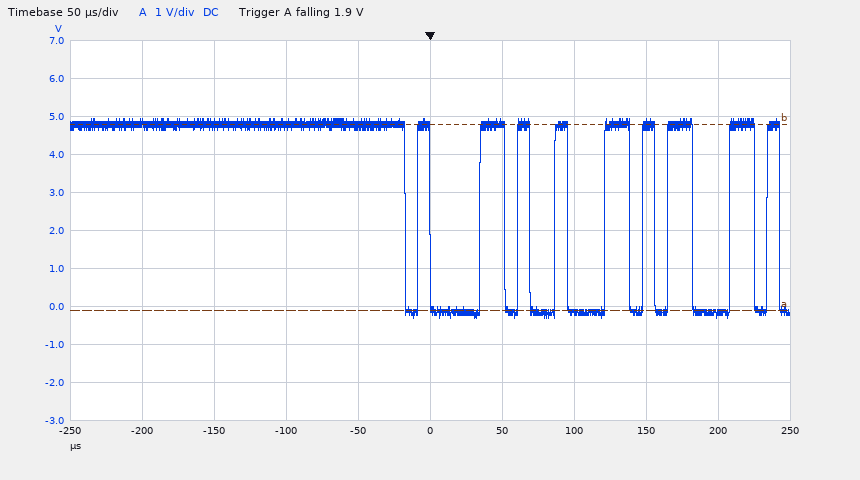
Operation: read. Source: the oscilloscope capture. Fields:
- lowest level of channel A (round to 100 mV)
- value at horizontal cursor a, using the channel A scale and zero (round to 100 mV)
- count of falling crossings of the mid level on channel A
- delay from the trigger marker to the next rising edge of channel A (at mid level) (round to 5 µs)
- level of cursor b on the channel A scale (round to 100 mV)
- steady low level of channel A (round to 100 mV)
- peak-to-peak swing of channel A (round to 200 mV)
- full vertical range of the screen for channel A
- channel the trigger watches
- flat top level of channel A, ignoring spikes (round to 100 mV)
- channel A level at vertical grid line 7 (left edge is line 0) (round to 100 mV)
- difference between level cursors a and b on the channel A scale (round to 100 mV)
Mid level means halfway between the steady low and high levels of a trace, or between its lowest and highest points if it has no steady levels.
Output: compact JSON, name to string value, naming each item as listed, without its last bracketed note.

{"lowest level of channel A": "-300 mV", "value at horizontal cursor a, using the channel A scale and zero": "-100 mV", "count of falling crossings of the mid level on channel A": "10", "delay from the trigger marker to the next rising edge of channel A (at mid level)": "35 µs", "level of cursor b on the channel A scale": "4.8 V", "steady low level of channel A": "-200 mV", "peak-to-peak swing of channel A": "5.2 V", "full vertical range of the screen for channel A": "10 V", "channel the trigger watches": "channel A", "flat top level of channel A, ignoring spikes": "4.8 V", "channel A level at vertical grid line 7 (left edge is line 0)": "-200 mV", "difference between level cursors a and b on the channel A scale": "4.9 V"}
